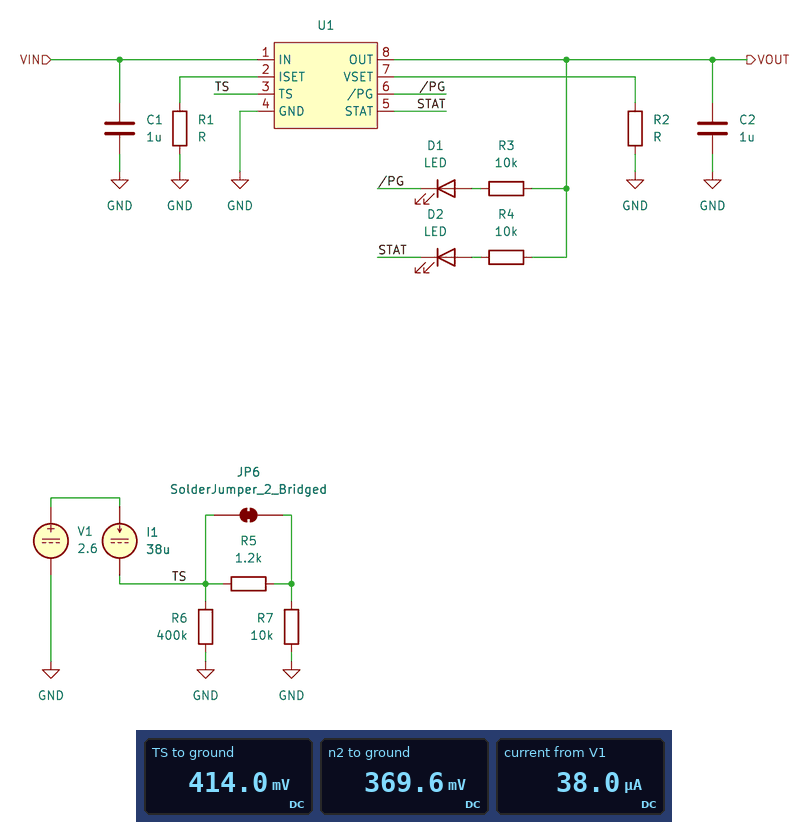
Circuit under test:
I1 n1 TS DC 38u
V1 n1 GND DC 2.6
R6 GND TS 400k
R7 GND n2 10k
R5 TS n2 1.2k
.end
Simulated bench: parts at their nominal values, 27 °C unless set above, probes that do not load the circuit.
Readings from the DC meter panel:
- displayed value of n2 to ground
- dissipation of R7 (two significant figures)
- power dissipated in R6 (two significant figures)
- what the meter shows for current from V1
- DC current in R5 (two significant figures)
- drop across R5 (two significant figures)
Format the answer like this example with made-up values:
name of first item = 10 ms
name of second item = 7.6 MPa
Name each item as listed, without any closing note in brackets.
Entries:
displayed value of n2 to ground = 369.6 mV
dissipation of R7 = 14 µW
power dissipated in R6 = 430 nW
what the meter shows for current from V1 = 38.0 µA
DC current in R5 = 37 µA
drop across R5 = 44 mV
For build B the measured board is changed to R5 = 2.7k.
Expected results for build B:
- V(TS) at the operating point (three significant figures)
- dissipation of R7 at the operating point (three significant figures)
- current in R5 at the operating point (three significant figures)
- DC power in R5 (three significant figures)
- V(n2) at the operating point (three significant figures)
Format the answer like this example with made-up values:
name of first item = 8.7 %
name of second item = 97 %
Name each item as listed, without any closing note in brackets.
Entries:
V(TS) at the operating point = 468 mV
dissipation of R7 at the operating point = 13.6 µW
current in R5 at the operating point = 36.8 µA
DC power in R5 = 3.66 µW
V(n2) at the operating point = 368 mV
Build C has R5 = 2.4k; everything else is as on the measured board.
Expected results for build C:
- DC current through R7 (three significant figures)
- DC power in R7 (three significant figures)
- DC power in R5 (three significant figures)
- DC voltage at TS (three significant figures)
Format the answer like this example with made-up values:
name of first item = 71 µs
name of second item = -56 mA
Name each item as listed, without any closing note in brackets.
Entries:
DC current through R7 = 36.9 µA
DC power in R7 = 13.6 µW
DC power in R5 = 3.26 µW
DC voltage at TS = 457 mV
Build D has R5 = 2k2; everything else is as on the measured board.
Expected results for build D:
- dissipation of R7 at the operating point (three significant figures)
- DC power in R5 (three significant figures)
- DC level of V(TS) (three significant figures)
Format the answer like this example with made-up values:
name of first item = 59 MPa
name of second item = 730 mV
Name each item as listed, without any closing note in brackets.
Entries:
dissipation of R7 at the operating point = 13.6 µW
DC power in R5 = 2.99 µW
DC level of V(TS) = 450 mV
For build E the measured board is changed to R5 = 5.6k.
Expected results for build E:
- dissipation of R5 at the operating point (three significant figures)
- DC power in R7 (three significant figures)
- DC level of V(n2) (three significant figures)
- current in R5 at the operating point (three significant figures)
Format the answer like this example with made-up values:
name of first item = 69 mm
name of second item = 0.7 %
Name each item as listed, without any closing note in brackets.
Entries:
dissipation of R5 at the operating point = 7.49 µW
DC power in R7 = 13.4 µW
DC level of V(n2) = 366 mV
current in R5 at the operating point = 36.6 µA
